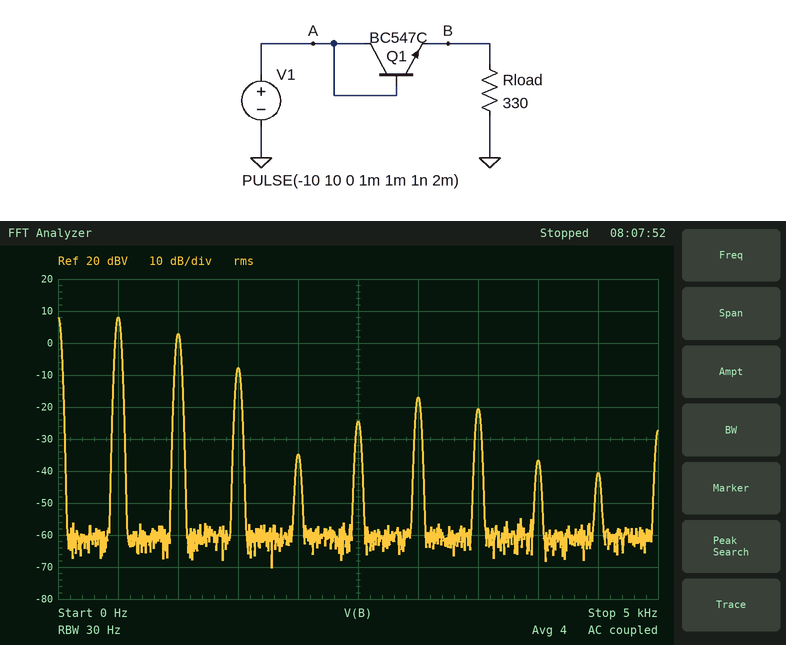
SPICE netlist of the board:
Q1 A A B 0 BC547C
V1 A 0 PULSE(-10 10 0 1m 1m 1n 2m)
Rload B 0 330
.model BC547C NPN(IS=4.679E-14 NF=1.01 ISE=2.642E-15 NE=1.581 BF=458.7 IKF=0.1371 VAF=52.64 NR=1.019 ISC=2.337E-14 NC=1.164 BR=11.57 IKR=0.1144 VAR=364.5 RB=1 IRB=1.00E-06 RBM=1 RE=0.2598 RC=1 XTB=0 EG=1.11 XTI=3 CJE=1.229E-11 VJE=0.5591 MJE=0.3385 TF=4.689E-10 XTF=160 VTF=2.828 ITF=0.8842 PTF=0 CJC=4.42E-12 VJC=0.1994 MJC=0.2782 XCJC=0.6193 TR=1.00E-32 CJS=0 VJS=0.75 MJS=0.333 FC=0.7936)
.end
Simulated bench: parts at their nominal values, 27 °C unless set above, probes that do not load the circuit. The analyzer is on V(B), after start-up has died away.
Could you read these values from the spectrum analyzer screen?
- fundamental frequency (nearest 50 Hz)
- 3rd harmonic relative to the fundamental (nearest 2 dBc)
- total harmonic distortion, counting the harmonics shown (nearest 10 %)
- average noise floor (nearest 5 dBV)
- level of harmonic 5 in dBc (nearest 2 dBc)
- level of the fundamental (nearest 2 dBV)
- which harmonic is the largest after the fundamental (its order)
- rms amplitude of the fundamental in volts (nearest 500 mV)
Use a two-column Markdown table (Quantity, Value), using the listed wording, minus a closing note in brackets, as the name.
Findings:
| Quantity | Value |
|---|---|
| fundamental frequency | 500 Hz |
| 3rd harmonic relative to the fundamental | -16 dBc |
| total harmonic distortion, counting the harmonics shown | 60 % |
| average noise floor | -60 dBV |
| level of harmonic 5 in dBc | -32 dBc |
| level of the fundamental | 8 dBV |
| which harmonic is the largest after the fundamental | 2 |
| rms amplitude of the fundamental in volts | 2.5 V |
